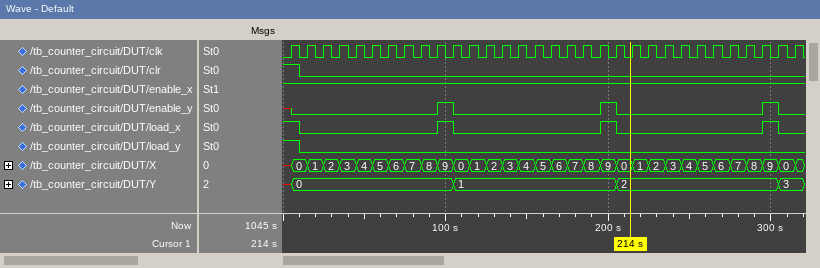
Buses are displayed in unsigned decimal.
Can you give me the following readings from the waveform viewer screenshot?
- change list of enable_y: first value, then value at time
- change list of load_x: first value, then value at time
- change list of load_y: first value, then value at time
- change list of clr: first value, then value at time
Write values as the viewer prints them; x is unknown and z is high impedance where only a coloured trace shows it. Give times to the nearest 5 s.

x, 0 at 5 s, 1 at 95 s, 0 at 105 s, 1 at 195 s, 0 at 205 s, 1 at 295 s, 0 at 305 s
1, 0 at 10 s, 1 at 95 s, 0 at 105 s, 1 at 195 s, 0 at 205 s, 1 at 295 s, 0 at 305 s
1, 0 at 10 s
1, 0 at 10 s
